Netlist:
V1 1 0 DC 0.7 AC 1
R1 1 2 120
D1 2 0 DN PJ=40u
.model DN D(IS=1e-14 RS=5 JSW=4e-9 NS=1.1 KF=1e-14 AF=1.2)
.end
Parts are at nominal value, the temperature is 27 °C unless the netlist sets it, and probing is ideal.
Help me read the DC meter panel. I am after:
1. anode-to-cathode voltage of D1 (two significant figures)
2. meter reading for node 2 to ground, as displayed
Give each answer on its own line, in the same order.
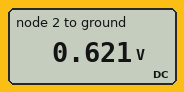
620 mV
0.621 V
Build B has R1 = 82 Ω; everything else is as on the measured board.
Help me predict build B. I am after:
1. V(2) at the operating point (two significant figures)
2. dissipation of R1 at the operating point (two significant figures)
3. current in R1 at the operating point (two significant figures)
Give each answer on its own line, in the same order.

630 mV
61 µW
860 µA
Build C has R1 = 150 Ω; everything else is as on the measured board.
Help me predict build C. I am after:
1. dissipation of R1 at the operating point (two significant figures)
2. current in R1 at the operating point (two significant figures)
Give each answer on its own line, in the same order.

47 µW
560 µA
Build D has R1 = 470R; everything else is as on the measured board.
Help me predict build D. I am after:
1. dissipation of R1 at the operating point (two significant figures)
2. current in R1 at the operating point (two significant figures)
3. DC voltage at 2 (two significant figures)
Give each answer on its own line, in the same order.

26 µW
230 µA
590 mV
